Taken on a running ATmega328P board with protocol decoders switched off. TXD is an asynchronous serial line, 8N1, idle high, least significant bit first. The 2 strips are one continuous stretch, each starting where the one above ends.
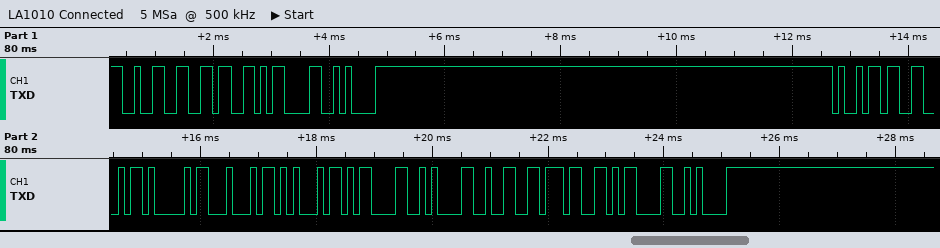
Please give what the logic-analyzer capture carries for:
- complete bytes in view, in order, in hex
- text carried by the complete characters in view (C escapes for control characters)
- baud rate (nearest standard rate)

0x32 0x36 0x0D 0x0A 0x69 0x46 0x41 0x44 0x45 0x0D 0x0A 0x32 0x37 0x0D 0x0A
"26\r\niFADE\r\n27\r\n"
9600 baud
